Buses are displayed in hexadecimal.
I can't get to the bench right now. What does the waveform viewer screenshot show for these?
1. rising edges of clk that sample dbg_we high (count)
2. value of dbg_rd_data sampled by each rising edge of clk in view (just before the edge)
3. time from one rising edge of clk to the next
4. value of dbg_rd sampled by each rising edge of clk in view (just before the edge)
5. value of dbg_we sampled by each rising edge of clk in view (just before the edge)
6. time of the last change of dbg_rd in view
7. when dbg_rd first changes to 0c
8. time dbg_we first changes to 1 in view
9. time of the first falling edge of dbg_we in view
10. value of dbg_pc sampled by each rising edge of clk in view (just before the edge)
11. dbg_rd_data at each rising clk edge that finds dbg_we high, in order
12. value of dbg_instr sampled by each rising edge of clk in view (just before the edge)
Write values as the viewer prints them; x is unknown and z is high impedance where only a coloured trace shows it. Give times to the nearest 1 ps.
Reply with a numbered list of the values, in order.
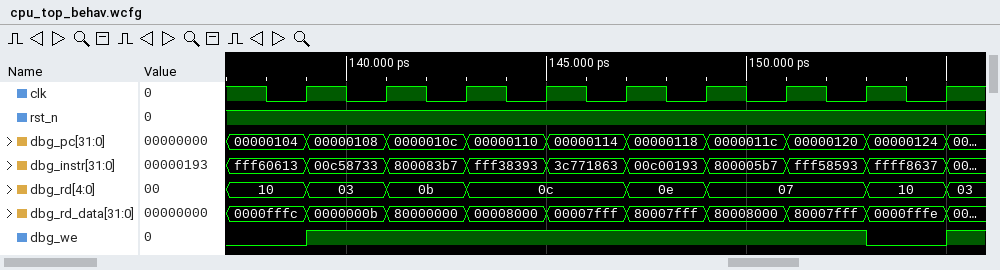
1. 7
2. 0000fffc, 0000000b, 80000000, 00008000, 00007fff, 80007fff, 80008000, 80007fff, 0000fffe
3. 2 ps
4. 10, 03, 0b, 0c, 0c, 0e, 07, 07, 10
5. 0 1 1 1 1 1 1 1 0
6. 155 ps
7. 143 ps
8. 139 ps
9. 153 ps
10. 00000104, 00000108, 0000010c, 00000110, 00000114, 00000118, 0000011c, 00000120, 00000124
11. 0000000b, 80000000, 00008000, 00007fff, 80007fff, 80008000, 80007fff
12. fff60613, 00c58733, 800083b7, fff38393, 3c771863, 00c00193, 800005b7, fff58593, ffff8637
